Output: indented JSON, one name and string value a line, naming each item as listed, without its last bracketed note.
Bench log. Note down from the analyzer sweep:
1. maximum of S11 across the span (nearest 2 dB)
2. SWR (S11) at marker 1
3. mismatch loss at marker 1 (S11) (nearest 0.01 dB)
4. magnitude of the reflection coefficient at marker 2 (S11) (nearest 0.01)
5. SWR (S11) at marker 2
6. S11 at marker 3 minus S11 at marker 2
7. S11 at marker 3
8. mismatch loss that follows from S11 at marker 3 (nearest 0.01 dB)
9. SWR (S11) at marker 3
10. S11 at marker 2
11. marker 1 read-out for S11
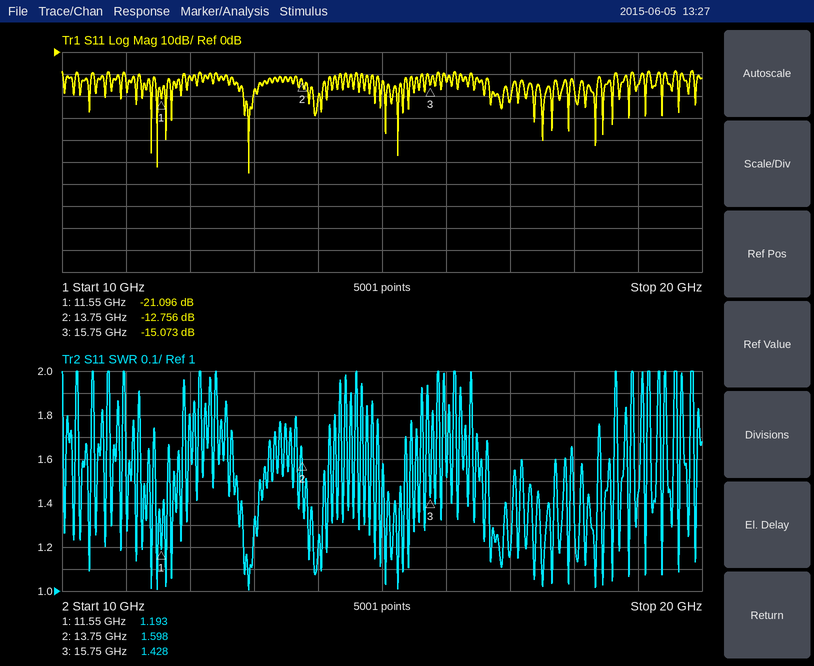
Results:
{
  "maximum of S11 across the span": "-8 dB",
  "SWR (S11) at marker 1": "1.193",
  "mismatch loss at marker 1 (S11)": "0.03 dB",
  "magnitude of the reflection coefficient at marker 2 (S11)": "0.23",
  "SWR (S11) at marker 2": "1.598",
  "S11 at marker 3 minus S11 at marker 2": "-2.317 dB",
  "S11 at marker 3": "-15.073 dB",
  "mismatch loss that follows from S11 at marker 3": "0.14 dB",
  "SWR (S11) at marker 3": "1.428",
  "S11 at marker 2": "-12.756 dB",
  "marker 1 read-out for S11": "-21.096 dB"
}
